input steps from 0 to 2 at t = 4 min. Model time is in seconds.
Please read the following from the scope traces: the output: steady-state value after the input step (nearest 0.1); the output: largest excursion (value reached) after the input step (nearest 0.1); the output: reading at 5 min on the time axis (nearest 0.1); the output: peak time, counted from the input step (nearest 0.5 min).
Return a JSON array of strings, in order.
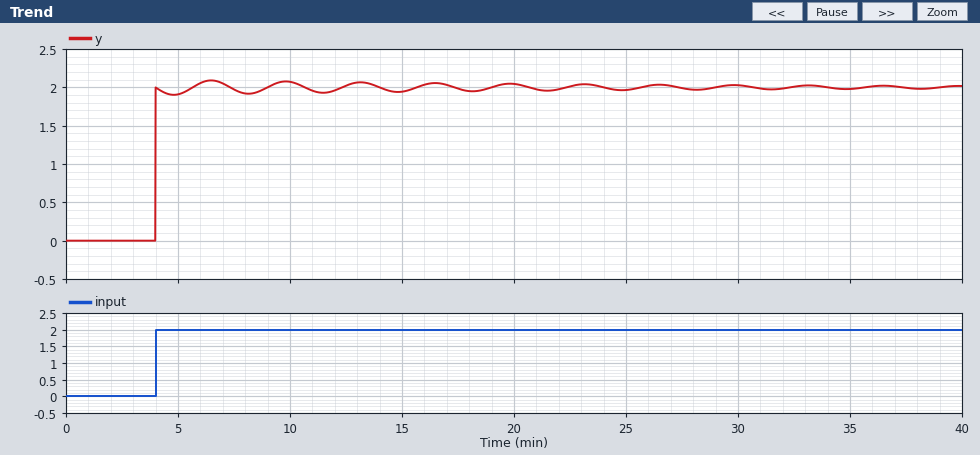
["2.0", "2.1", "1.9", "2.5 min"]
